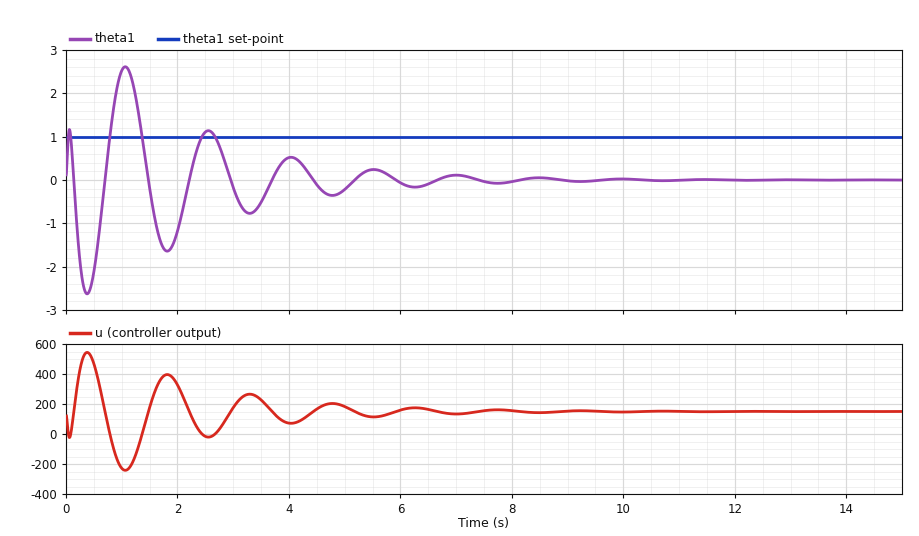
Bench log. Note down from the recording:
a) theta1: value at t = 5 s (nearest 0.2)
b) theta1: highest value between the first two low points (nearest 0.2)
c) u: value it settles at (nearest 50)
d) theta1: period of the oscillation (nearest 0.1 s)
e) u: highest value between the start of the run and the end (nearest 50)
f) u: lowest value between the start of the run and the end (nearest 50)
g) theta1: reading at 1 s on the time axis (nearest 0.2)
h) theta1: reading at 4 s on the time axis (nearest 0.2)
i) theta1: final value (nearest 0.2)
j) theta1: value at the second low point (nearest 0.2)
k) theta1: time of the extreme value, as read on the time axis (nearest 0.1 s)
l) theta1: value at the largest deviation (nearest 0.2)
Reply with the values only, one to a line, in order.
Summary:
-0.2
2.6
150
1.4 s
550
-250
2.6
0.6
0.0
-1.6
0.4 s
-2.6
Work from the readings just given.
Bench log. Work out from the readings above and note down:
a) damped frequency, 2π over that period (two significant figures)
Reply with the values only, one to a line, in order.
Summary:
4.5 rad/s
